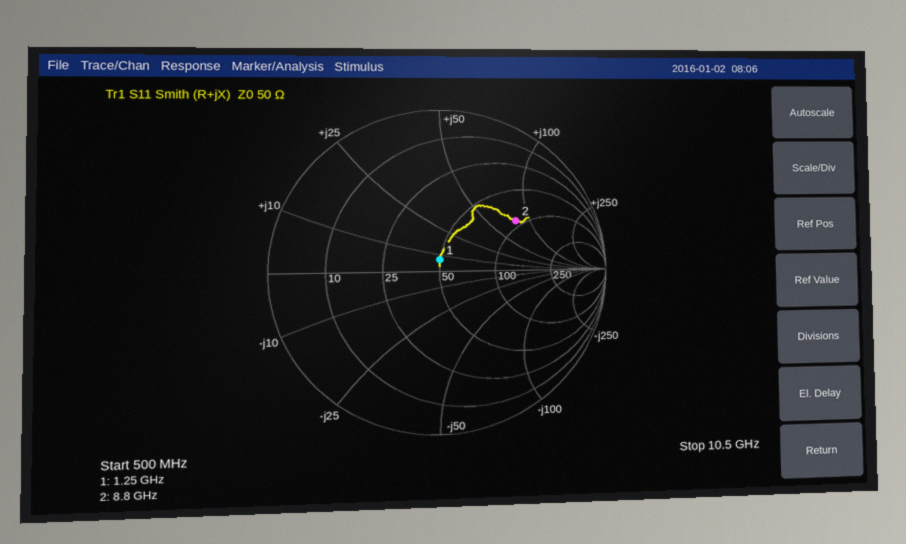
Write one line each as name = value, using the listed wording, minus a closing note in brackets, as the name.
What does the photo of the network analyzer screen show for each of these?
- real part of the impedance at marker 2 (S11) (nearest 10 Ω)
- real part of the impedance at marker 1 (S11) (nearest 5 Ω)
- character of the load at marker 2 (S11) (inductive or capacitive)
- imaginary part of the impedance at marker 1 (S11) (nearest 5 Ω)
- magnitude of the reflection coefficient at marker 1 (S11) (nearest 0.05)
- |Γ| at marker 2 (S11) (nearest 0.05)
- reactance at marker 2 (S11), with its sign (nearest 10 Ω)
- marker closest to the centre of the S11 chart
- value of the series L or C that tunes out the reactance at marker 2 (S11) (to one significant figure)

real part of the impedance at marker 2 (S11) = 90 Ω
real part of the impedance at marker 1 (S11) = 50 Ω
character of the load at marker 2 (S11) = inductive
imaginary part of the impedance at marker 1 (S11) = +5 Ω
magnitude of the reflection coefficient at marker 1 (S11) = 0.05
|Γ| at marker 2 (S11) = 0.55
reactance at marker 2 (S11), with its sign = +80 Ω
marker closest to the centre of the S11 chart = marker 1
value of the series L or C that tunes out the reactance at marker 2 (S11) = 200 fF
